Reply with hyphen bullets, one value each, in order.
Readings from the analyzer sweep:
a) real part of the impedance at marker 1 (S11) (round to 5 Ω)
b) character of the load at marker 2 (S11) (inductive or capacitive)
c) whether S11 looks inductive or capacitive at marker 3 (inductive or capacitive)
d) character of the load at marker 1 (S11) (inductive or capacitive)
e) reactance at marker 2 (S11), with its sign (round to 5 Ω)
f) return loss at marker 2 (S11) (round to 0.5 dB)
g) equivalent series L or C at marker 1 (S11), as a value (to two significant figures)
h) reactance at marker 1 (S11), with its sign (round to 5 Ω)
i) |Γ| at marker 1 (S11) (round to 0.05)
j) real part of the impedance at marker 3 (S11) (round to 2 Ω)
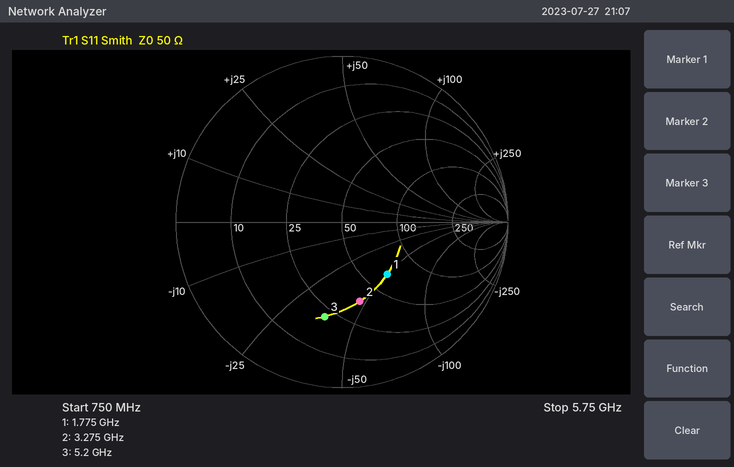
- 65 Ω
- capacitive
- capacitive
- capacitive
- -45 Ω
- 6.0 dB
- 1.8 pF
- -50 Ω
- 0.40
- 22 Ω
